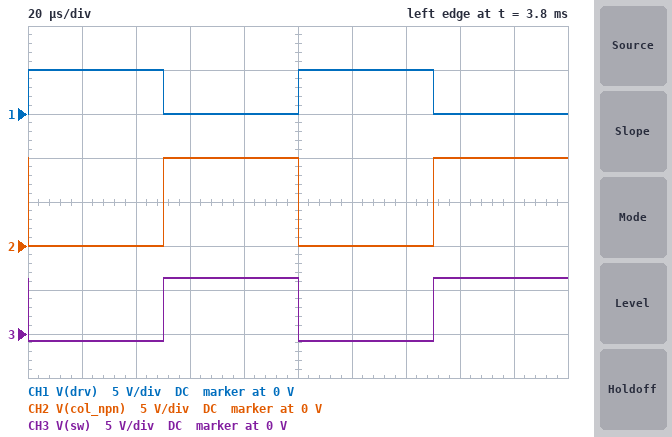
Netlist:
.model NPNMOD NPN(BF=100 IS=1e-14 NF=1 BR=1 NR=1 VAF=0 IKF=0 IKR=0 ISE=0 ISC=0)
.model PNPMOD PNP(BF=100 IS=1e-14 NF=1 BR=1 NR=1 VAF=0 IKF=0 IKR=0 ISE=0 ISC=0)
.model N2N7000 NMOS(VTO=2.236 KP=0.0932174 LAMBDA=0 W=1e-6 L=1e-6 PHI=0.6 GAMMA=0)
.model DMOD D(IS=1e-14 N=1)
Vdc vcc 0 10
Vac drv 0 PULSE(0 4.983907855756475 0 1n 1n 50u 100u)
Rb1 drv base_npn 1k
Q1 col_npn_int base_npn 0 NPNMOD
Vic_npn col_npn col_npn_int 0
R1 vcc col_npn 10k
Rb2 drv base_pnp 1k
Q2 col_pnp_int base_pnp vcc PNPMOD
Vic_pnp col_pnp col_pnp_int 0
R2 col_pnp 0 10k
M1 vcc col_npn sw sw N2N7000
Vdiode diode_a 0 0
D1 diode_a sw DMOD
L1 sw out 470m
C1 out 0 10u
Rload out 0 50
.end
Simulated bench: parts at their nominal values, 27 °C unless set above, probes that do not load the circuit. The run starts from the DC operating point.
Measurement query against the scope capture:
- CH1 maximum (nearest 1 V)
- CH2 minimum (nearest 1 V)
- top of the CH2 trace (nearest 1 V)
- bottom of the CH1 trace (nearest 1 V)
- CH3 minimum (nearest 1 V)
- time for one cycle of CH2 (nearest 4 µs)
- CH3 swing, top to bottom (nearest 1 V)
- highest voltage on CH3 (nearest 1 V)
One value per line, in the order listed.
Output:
5 V
0 V
10 V
0 V
-1 V
100 µs
7 V
6 V
